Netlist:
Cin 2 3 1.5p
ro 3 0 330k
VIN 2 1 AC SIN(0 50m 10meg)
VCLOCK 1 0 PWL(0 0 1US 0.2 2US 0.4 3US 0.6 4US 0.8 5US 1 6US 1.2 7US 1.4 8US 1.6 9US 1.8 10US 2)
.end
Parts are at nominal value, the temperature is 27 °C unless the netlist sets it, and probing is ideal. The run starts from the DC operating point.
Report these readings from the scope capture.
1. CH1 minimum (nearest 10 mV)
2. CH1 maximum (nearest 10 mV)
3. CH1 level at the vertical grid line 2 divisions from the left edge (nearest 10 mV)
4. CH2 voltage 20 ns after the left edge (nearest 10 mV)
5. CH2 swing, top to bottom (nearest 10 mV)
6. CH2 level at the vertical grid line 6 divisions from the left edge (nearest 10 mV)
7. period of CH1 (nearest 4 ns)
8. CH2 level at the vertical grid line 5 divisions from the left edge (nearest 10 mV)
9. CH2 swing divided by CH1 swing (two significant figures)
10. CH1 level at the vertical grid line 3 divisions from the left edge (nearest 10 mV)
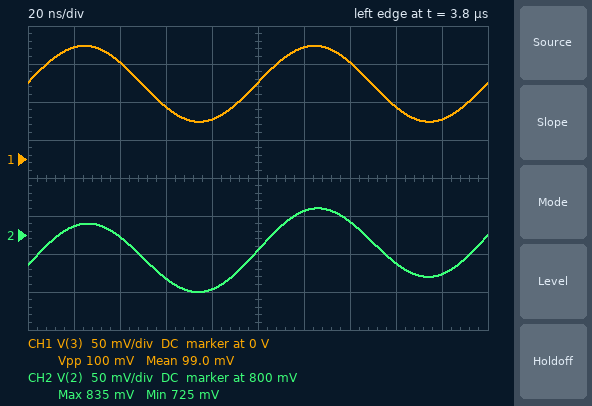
50 mV
150 mV
130 mV
810 mV
110 mV
830 mV
100 ns
780 mV
1.1
70 mV
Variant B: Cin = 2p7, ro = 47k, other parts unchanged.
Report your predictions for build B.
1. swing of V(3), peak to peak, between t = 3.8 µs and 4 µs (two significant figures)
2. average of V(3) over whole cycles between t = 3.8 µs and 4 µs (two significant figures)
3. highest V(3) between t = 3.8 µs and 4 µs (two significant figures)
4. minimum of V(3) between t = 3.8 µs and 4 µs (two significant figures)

99 mV
25 mV
75 mV
-24 mV
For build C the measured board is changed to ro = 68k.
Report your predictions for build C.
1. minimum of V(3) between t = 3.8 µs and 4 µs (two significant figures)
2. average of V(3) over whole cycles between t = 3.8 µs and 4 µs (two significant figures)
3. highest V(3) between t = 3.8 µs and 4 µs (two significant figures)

-29 mV
20 mV
70 mV
